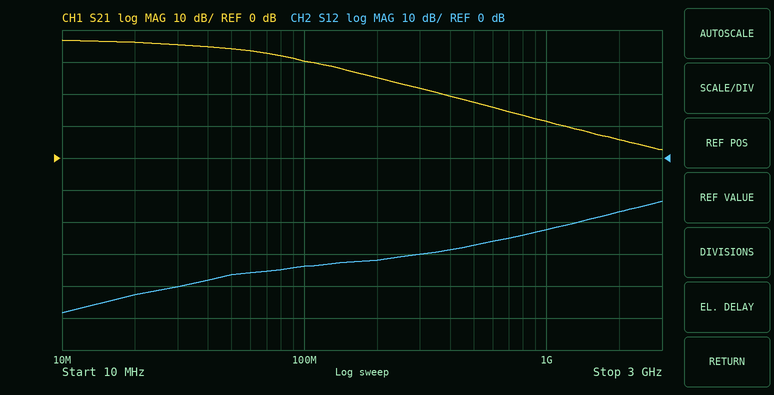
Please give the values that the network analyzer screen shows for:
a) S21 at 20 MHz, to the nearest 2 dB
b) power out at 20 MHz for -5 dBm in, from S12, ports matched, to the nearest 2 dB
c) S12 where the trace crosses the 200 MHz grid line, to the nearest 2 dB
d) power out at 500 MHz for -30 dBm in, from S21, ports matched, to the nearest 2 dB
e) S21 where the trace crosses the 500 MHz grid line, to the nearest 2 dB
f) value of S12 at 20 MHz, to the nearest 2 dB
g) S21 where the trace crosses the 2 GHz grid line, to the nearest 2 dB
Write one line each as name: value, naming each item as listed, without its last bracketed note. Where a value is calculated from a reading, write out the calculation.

S21 at 20 MHz, to the nearest 2 dB: 36 dB
power out at 20 MHz for -5 dBm in, from S12, ports matched, to the nearest 2 dB: -5 dBm + (-42 dB) = -48 dBm
S12 where the trace crosses the 200 MHz grid line, to the nearest 2 dB: -32 dB
power out at 500 MHz for -30 dBm in, from S21, ports matched, to the nearest 2 dB: -30 dBm + (18 dB) = -12 dBm
S21 where the trace crosses the 500 MHz grid line, to the nearest 2 dB: 18 dB
value of S12 at 20 MHz, to the nearest 2 dB: -42 dB
S21 where the trace crosses the 2 GHz grid line, to the nearest 2 dB: 6 dB
